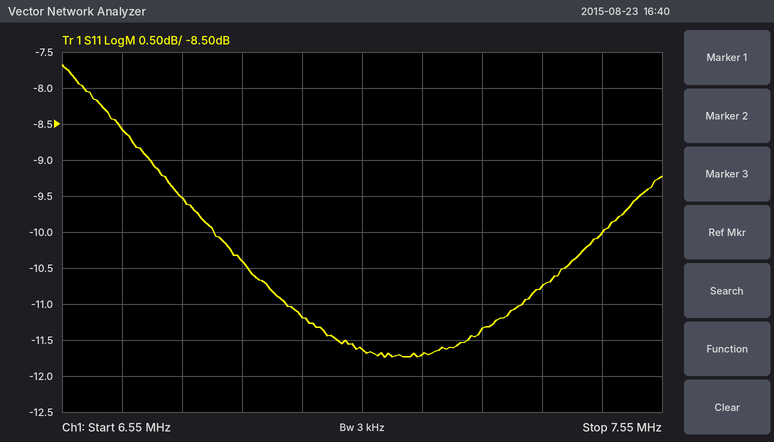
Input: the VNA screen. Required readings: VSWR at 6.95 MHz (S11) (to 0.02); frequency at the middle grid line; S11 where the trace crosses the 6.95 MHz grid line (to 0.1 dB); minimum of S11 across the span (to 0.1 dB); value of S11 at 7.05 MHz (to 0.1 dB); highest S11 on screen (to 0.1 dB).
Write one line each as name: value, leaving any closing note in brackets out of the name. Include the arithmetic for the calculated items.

VSWR at 6.95 MHz (S11): |Γ| = 10^(-11.2/20) = 0.2754; VSWR = (1 + 0.2754)/(1 − 0.2754) ≈ 1.76
frequency at the middle grid line: 7.05 MHz
S11 where the trace crosses the 6.95 MHz grid line: -11.2 dB
minimum of S11 across the span: -11.7 dB
value of S11 at 7.05 MHz: -11.6 dB
highest S11 on screen: -7.7 dB
